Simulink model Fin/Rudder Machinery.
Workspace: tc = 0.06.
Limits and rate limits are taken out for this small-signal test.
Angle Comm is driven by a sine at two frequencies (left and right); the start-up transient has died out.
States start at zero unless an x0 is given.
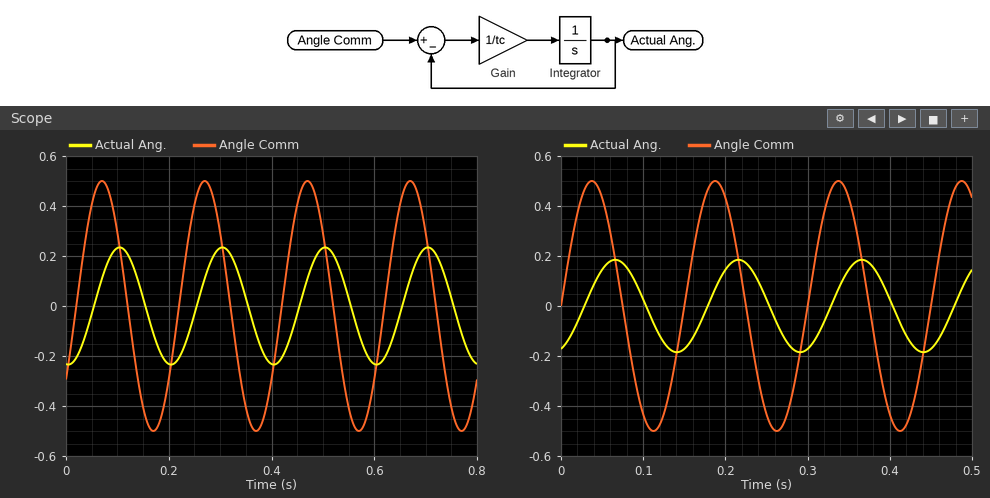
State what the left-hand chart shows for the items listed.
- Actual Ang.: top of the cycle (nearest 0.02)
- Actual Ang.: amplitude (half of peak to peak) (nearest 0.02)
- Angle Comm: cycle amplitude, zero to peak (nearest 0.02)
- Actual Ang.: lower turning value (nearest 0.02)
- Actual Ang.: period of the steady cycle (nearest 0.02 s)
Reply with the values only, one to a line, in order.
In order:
0.24
0.24
0.50
-0.24
0.20 s
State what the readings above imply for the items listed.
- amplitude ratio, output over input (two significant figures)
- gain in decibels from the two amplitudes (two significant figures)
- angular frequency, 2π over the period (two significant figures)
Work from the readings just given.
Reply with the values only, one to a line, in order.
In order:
0.48
-6.4 dB
31 rad/s
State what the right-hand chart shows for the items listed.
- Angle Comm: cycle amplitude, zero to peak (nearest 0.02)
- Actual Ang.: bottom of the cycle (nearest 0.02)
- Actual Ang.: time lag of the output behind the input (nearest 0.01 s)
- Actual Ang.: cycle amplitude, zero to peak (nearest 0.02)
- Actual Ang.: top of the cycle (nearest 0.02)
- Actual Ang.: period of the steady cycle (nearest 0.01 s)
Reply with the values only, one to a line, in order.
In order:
0.50
-0.18
0.03 s
0.18
0.18
0.15 s
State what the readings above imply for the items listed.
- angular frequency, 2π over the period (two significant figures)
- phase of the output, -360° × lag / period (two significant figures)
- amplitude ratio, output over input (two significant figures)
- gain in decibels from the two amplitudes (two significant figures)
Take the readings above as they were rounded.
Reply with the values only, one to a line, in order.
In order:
42 rad/s
-72°
0.36
-8.9 dB
